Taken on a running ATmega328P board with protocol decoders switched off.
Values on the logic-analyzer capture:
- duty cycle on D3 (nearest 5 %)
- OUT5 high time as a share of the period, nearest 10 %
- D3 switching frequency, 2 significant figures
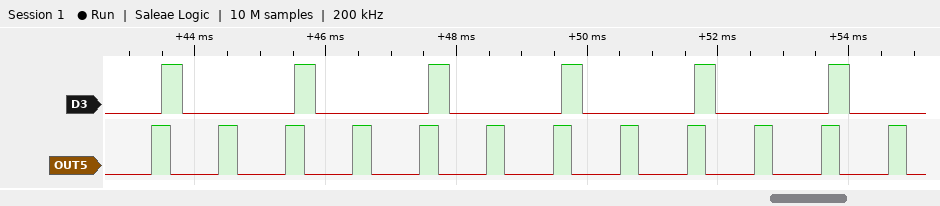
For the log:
15 %
30 %
490 Hz
